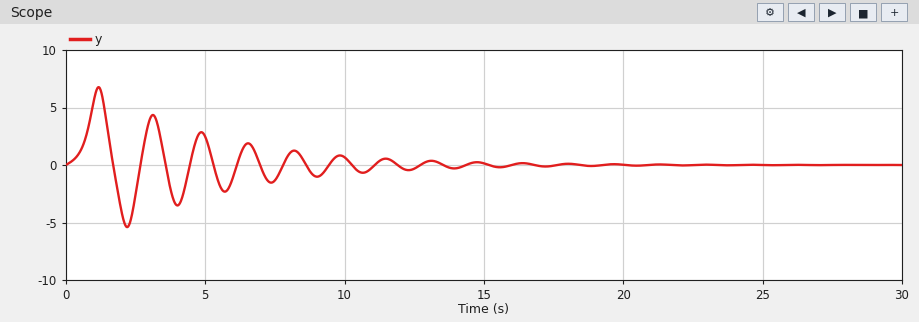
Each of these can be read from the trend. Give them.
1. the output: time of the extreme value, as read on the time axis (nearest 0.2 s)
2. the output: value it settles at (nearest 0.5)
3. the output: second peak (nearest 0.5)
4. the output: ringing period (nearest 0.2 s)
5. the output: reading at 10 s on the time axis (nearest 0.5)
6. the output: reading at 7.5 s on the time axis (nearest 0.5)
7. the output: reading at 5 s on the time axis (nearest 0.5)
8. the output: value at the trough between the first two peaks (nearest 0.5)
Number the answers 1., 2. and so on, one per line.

1. 1.2 s
2. 0.0
3. 4.5
4. 2.0 s
5. 0.5
6. -1.5
7. 2.5
8. -5.5
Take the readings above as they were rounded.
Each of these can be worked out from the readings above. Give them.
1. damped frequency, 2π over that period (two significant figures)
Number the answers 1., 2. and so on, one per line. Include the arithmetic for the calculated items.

1. 2π / 2 = 3.1 rad/s
